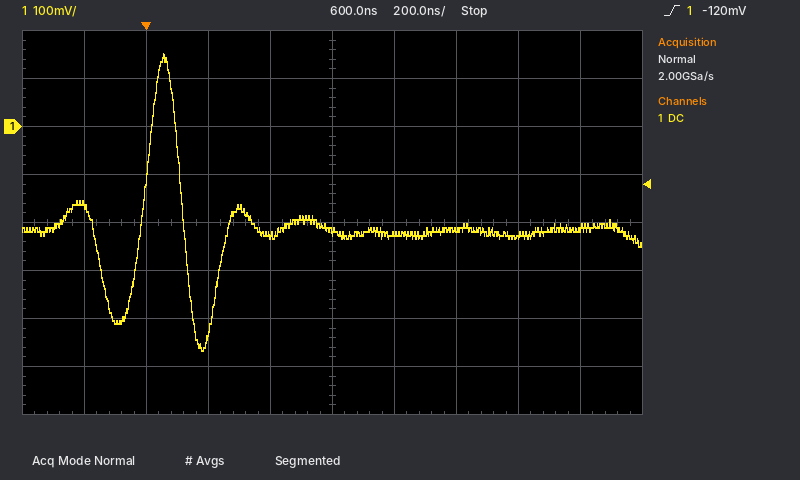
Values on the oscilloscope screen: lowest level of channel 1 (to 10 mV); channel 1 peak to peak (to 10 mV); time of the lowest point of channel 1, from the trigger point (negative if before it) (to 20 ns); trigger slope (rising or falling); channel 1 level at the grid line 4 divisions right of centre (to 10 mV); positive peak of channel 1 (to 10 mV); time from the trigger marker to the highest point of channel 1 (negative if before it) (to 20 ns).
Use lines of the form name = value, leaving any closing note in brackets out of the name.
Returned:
lowest level of channel 1 = -470 mV
channel 1 peak to peak = 620 mV
time of the lowest point of channel 1, from the trigger point (negative if before it) = +180 ns
trigger slope = rising
channel 1 level at the grid line 4 divisions right of centre = -210 mV
positive peak of channel 1 = 150 mV
time from the trigger marker to the highest point of channel 1 (negative if before it) = +60 ns
